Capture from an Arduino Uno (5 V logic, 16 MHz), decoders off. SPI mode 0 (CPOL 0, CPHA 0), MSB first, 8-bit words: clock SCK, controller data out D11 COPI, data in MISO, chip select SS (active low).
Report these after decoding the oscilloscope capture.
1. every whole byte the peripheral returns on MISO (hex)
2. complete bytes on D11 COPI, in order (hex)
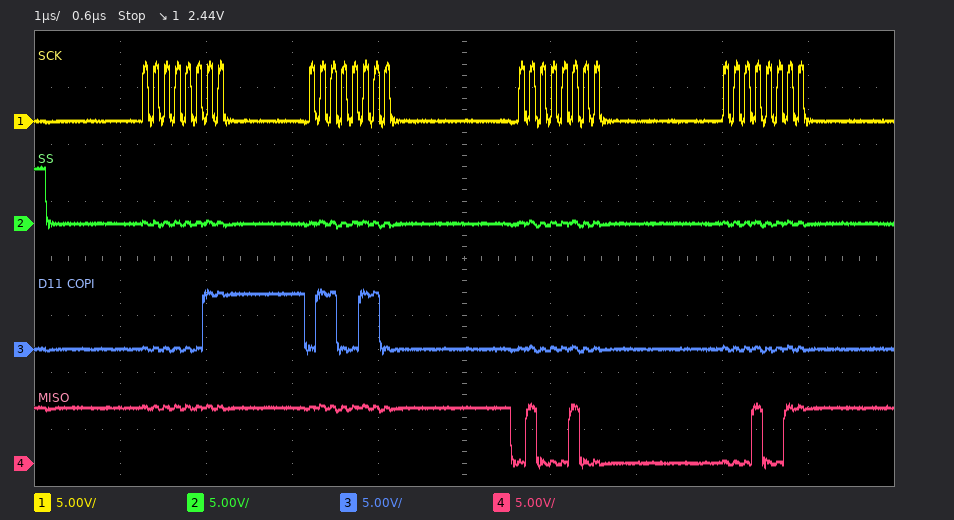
0xFF 0xFF 0x44 0x13
0x03 0x66 0x00 0x00
